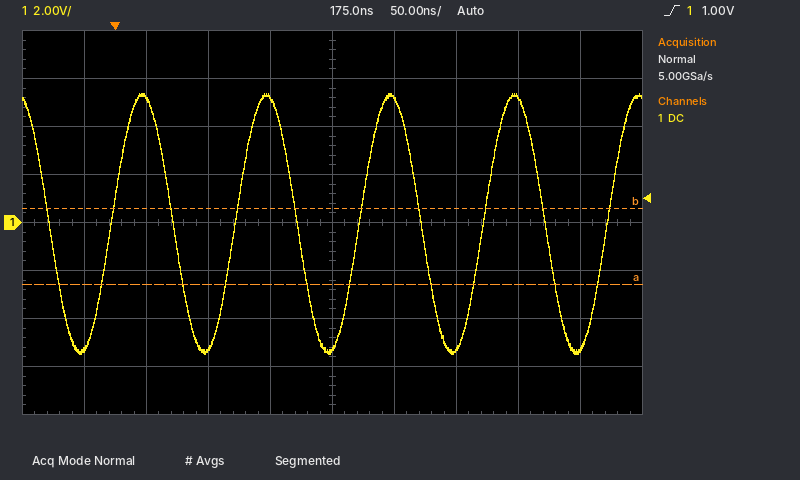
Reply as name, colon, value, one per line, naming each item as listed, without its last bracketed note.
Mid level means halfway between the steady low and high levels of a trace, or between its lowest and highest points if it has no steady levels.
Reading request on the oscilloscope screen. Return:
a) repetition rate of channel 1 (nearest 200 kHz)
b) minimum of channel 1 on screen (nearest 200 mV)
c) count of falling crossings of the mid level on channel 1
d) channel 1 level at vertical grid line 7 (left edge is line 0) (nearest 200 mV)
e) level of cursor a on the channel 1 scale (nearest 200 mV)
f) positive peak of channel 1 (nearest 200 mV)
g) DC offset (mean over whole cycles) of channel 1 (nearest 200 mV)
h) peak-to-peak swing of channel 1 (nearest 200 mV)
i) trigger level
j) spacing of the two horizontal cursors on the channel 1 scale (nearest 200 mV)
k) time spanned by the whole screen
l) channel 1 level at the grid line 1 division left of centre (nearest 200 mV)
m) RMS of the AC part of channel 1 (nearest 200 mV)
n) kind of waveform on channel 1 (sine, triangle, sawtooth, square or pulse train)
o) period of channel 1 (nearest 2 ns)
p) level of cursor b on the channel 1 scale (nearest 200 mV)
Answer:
repetition rate of channel 1: 10.0 MHz
minimum of channel 1 on screen: -5.4 V
count of falling crossings of the mid level on channel 1: 5
channel 1 level at vertical grid line 7 (left edge is line 0): -5.2 V
level of cursor a on the channel 1 scale: -2.6 V
positive peak of channel 1: 5.4 V
DC offset (mean over whole cycles) of channel 1: 0.0 V
peak-to-peak swing of channel 1: 10.8 V
trigger level: 1.00 V
spacing of the two horizontal cursors on the channel 1 scale: 3.2 V
time spanned by the whole screen: 500 ns
channel 1 level at the grid line 1 division left of centre: 5.2 V
RMS of the AC part of channel 1: 3.8 V
kind of waveform on channel 1: sine
period of channel 1: 100 ns
level of cursor b on the channel 1 scale: 600 mV
